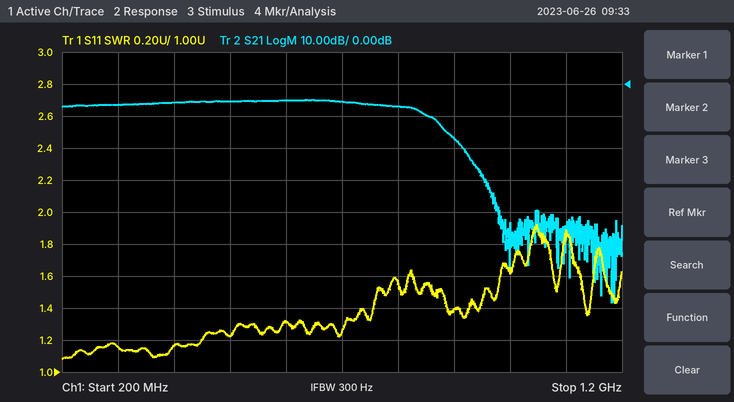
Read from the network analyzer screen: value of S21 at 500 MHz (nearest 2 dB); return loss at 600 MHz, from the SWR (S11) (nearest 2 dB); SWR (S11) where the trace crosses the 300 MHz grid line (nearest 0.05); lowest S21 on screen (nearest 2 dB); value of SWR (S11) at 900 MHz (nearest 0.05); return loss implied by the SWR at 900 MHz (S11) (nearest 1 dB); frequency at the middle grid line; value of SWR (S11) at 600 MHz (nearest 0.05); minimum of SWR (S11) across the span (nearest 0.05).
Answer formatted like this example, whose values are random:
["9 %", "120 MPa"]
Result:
["-6 dB", "18 dB", "1.15", "-68 dB", "1.40", "16 dB", "700 MHz", "1.30", "1.10"]
